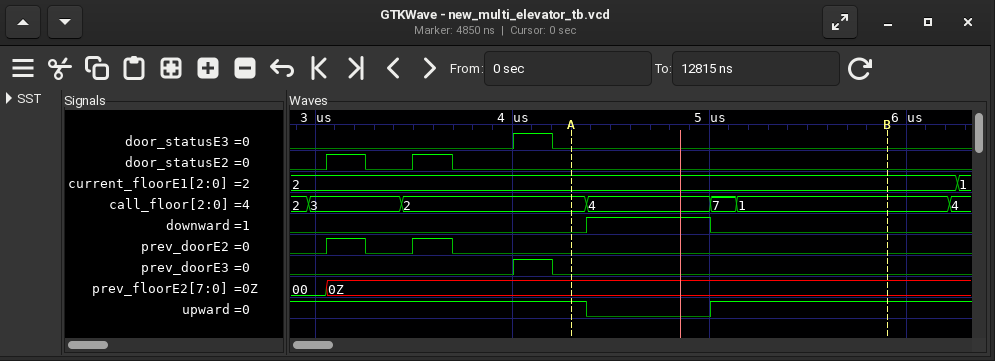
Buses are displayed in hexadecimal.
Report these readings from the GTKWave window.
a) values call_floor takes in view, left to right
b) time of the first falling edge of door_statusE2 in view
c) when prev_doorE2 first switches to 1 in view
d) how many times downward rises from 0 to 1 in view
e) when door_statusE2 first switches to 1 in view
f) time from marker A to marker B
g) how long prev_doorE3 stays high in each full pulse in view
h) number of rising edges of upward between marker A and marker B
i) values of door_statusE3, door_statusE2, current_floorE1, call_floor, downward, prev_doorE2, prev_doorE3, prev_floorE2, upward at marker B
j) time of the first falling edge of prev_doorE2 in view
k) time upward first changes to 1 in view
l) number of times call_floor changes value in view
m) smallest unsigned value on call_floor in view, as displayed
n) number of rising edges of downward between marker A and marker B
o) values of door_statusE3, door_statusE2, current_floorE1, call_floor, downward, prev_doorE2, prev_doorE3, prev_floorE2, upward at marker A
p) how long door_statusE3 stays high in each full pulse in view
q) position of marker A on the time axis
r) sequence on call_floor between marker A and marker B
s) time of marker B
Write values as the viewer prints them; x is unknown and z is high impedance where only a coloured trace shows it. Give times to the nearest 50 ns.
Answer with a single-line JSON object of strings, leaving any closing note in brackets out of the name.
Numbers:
{"values call_floor takes in view, left to right": "2, 3, 2, 4, 7, 1, 4", "time of the first falling edge of door_statusE2 in view": "3250 ns", "when prev_doorE2 first switches to 1 in view": "3050 ns", "how many times downward rises from 0 to 1 in view": "1", "when door_statusE2 first switches to 1 in view": "3050 ns", "time from marker A to marker B": "1600 ns", "how long prev_doorE3 stays high in each full pulse in view": "200 ns", "number of rising edges of upward between marker A and marker B": "1", "values of door_statusE3, door_statusE2, current_floorE1, call_floor, downward, prev_doorE2, prev_doorE3, prev_floorE2, upward at marker B": "door_statusE3=0, door_statusE2=0, current_floorE1=2, call_floor=1, downward=0, prev_doorE2=0, prev_doorE3=0, prev_floorE2=0Z, upward=1", "time of the first falling edge of prev_doorE2 in view": "3250 ns", "time upward first changes to 1 in view": "5000 ns", "number of times call_floor changes value in view": "6", "smallest unsigned value on call_floor in view, as displayed": "1", "number of rising edges of downward between marker A and marker B": "1", "values of door_statusE3, door_statusE2, current_floorE1, call_floor, downward, prev_doorE2, prev_doorE3, prev_floorE2, upward at marker A": "door_statusE3=0, door_statusE2=0, current_floorE1=2, call_floor=2, downward=0, prev_doorE2=0, prev_doorE3=0, prev_floorE2=0Z, upward=1", "how long door_statusE3 stays high in each full pulse in view": "200 ns", "position of marker A on the time axis": "4300 ns", "sequence on call_floor between marker A and marker B": "2, 4, 7, 1", "time of marker B": "5900 ns"}
